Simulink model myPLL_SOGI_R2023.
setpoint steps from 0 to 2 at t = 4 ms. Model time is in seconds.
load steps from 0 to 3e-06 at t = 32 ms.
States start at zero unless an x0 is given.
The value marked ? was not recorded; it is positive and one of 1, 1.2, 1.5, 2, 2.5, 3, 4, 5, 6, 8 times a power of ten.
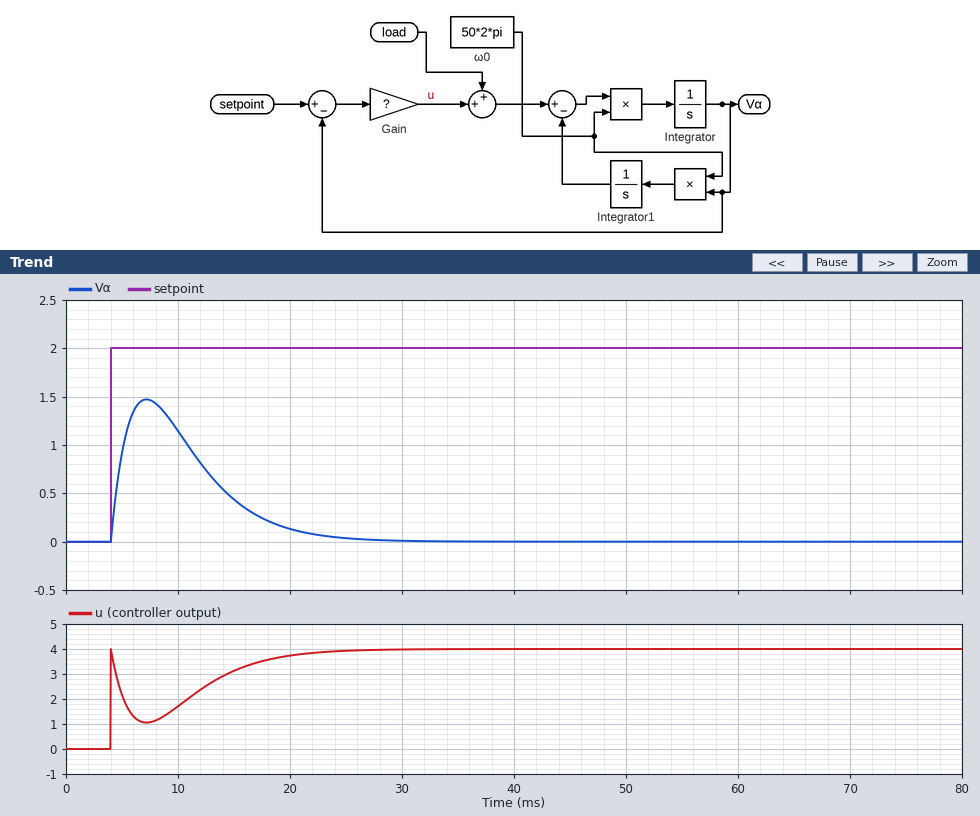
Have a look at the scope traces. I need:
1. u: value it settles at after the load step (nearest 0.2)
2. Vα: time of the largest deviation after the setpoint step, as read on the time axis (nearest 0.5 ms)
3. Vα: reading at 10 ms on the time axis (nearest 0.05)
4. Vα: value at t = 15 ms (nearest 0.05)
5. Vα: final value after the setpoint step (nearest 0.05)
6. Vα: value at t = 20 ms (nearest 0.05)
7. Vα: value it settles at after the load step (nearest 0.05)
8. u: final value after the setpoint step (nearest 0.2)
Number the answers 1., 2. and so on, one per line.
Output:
1. 4.0
2. 7.0 ms
3. 1.15
4. 0.45
5. 0.00
6. 0.15
7. 0.00
8. 4.0
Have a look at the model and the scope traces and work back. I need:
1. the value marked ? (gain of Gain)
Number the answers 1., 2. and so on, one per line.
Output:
1. 2
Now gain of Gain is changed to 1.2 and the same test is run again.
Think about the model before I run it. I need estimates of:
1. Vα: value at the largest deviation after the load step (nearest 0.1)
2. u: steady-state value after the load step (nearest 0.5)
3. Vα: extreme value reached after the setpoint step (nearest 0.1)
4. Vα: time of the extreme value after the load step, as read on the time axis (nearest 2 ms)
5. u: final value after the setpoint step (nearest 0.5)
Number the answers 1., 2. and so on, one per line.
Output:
1. 0.0
2. 2.5
3. 1.2
4. 46 ms
5. 2.5
